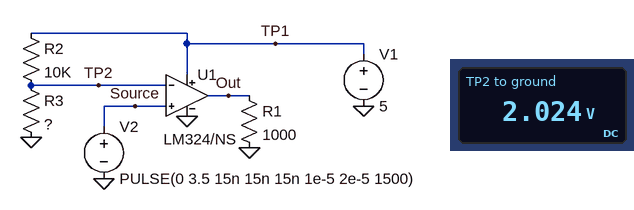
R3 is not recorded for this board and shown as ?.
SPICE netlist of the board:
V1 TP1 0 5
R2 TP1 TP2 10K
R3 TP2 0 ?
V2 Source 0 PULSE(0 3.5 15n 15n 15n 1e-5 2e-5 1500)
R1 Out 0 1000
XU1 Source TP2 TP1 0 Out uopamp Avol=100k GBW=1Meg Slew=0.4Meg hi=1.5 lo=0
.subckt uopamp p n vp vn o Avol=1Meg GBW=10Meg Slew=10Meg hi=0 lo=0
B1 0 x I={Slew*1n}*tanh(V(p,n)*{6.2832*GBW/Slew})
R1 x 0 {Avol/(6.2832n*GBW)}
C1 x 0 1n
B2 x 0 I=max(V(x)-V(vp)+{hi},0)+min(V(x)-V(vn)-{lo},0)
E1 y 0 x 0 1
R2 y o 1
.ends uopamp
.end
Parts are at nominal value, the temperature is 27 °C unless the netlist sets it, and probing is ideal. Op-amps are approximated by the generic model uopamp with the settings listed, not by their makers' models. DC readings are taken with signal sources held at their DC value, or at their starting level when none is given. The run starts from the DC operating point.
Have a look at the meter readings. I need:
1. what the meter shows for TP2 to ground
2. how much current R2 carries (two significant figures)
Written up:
2.024 V
300 µA
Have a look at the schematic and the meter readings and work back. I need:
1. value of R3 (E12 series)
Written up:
6.8 kΩ
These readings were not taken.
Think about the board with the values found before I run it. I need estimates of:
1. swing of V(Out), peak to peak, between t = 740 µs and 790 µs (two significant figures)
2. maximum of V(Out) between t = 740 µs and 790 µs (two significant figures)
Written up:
3.5 V
3.5 V
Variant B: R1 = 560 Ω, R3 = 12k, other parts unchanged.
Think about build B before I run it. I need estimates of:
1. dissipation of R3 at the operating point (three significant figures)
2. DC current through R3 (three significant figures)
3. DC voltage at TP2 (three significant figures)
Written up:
620 µW
227 µA
2.73 V
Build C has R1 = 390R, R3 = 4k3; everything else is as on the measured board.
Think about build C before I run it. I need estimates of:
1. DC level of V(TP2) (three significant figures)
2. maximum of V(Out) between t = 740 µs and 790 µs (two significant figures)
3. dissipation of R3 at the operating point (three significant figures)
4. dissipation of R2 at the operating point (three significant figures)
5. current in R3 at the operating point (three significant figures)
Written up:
1.50 V
3.5 V
526 µW
1.22 mW
350 µA
